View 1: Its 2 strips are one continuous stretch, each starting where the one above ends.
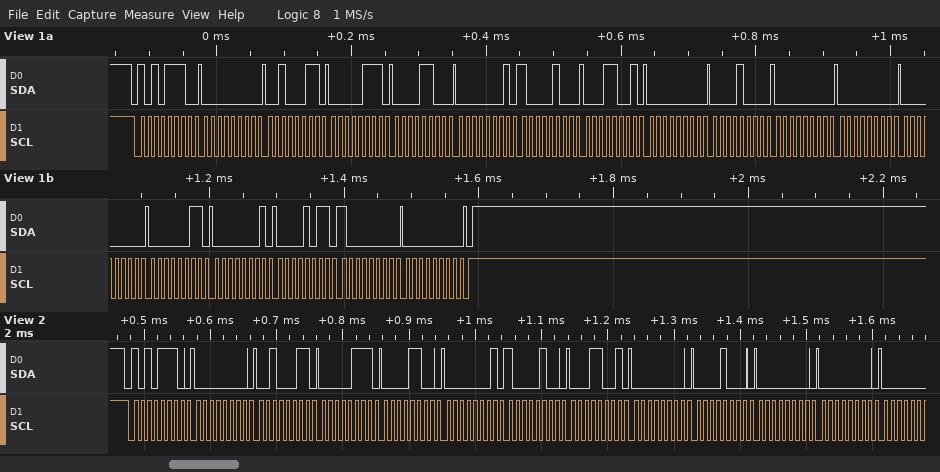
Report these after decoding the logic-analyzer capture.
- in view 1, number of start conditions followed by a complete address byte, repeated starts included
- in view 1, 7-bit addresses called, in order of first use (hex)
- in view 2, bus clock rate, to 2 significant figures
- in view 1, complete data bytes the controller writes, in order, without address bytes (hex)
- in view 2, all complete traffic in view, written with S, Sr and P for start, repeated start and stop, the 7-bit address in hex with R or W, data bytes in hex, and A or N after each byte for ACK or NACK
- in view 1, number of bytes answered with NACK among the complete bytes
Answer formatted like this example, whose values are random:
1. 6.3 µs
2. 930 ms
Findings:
1. 1
2. 0x57
3. 100 kHz
4. 00 23 07 0C 01 84 19 00 08 00 00 00 03 01 0B 80 00
5. S 57W A 00 A 23 A 07 A 0C A 01 A 84 A 19 A 00 A 08 A 00 A 00 A
6. 0
